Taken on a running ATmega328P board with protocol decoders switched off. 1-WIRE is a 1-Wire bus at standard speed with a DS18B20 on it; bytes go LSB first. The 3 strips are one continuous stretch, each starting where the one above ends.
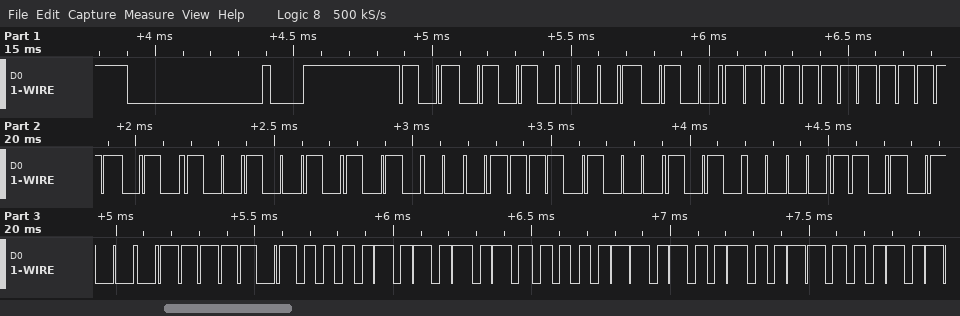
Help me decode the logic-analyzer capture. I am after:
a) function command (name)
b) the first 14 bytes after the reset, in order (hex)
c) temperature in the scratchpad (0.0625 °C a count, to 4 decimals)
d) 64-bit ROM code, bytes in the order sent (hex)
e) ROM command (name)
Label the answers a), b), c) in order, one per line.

a) Read Scratchpad
b) 55 28 FF 5F 49 85 17 05 2B BE 50 05 4B 46
c) 85.0000 °C
d) 28 FF 5F 49 85 17 05 2B
e) Match ROM
